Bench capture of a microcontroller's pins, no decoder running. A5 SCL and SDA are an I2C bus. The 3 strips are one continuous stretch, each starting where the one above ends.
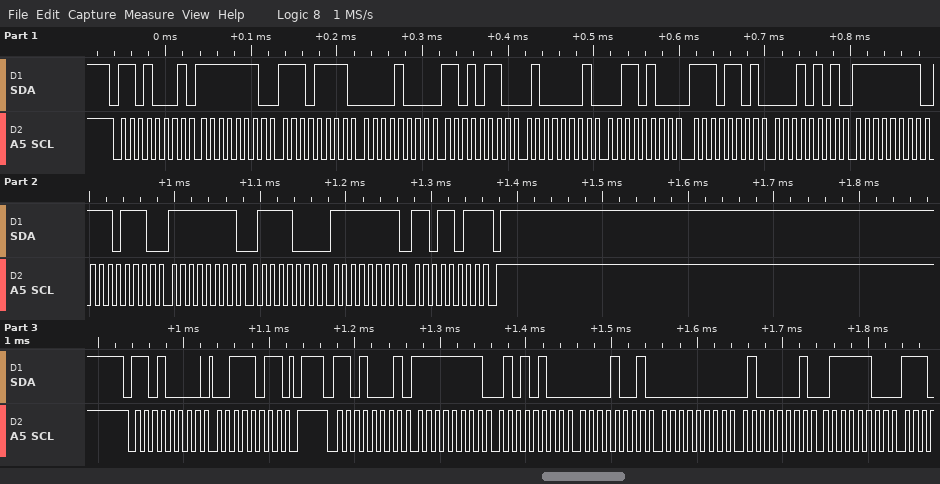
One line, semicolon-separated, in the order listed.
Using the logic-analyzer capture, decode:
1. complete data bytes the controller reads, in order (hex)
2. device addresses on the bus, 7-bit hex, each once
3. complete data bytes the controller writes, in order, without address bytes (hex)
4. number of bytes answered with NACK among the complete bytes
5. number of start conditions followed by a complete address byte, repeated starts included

FE EF 08 D6 41 34 ED 15 FF EE FF 78 FF DB FF 54 09 00 41 7C; 0x68; 3B; 1; 3
